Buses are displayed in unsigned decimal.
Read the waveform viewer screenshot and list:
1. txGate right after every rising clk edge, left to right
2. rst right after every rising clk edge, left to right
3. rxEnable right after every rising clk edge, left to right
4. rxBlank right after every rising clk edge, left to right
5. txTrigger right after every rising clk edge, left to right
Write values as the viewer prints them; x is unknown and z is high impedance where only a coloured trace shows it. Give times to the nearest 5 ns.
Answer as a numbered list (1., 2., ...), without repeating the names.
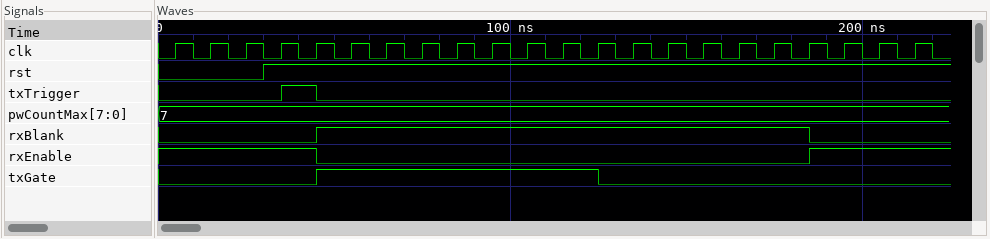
1. 0 0 0 0 1 1 1 1 1 1 1 1 0 0 0 0 0 0 0 0 0 0
2. 0 0 0 1 1 1 1 1 1 1 1 1 1 1 1 1 1 1 1 1 1 1
3. 1 1 1 1 0 0 0 0 0 0 0 0 0 0 0 0 0 0 1 1 1 1
4. 0 0 0 0 1 1 1 1 1 1 1 1 1 1 1 1 1 1 0 0 0 0
5. 0 0 0 1 0 0 0 0 0 0 0 0 0 0 0 0 0 0 0 0 0 0
